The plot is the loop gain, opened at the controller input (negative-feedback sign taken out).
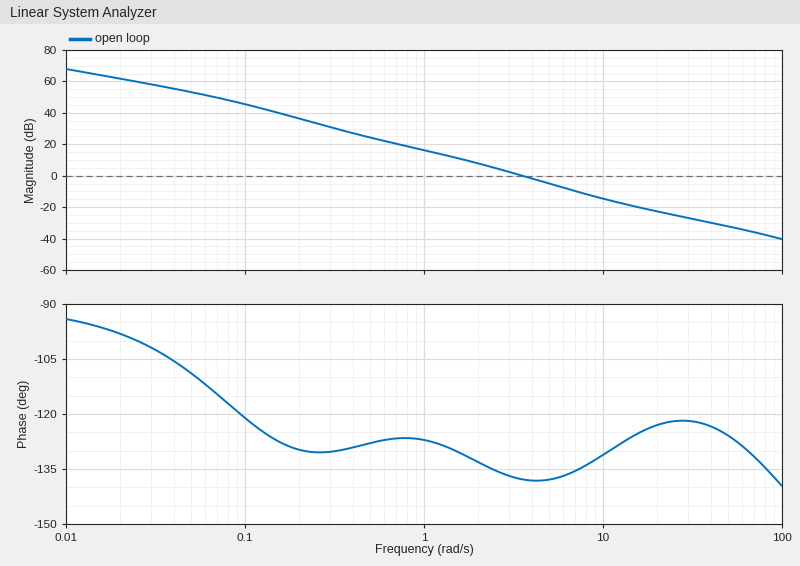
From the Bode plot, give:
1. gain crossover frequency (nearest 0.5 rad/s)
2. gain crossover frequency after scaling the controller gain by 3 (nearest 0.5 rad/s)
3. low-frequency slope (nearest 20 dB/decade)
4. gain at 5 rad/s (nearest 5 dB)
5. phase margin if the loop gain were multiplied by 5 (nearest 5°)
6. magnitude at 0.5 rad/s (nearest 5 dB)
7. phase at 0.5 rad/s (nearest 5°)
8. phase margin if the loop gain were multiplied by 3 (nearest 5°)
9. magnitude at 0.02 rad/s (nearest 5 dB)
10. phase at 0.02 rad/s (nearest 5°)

3.5 rad/s
7.0 rad/s
-20 dB/decade
-5 dB
50°
25 dB
-130°
45°
60 dB
-100°
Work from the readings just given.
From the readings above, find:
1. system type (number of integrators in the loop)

1
